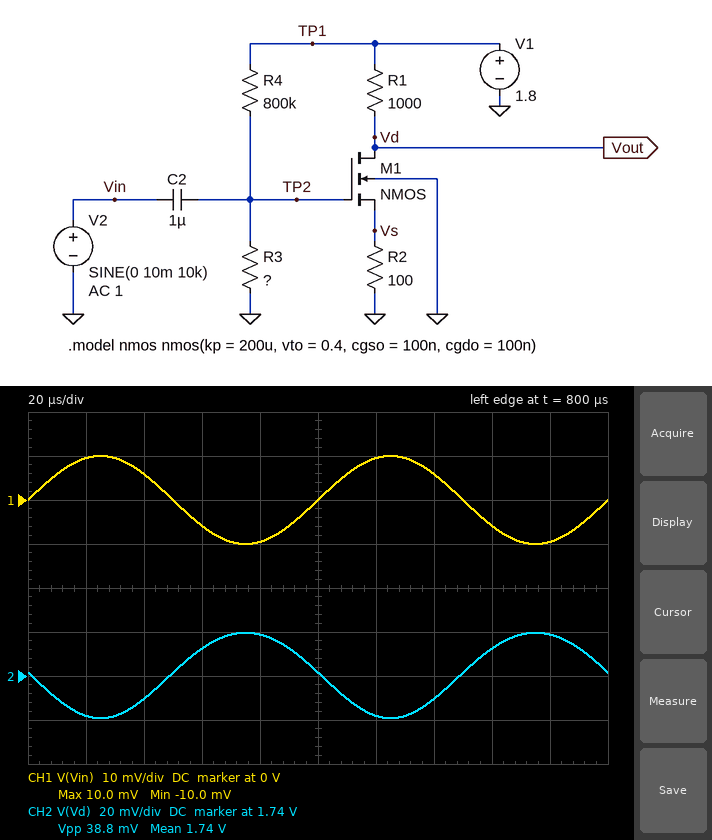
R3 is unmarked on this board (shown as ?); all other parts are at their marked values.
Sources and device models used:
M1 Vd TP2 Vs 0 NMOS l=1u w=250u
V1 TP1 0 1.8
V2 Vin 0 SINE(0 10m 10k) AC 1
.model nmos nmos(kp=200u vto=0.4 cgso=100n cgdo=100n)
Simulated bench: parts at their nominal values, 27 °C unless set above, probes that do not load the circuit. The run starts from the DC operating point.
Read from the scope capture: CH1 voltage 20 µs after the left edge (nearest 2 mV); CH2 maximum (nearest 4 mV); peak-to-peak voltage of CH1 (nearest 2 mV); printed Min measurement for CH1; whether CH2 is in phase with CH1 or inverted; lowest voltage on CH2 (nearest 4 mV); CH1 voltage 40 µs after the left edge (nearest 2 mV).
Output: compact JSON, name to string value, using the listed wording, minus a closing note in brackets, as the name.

{"CH1 voltage 20 µs after the left edge": "10 mV", "CH2 maximum": "1.760 V", "peak-to-peak voltage of CH1": "20 mV", "printed Min measurement for CH1": "-10.0 mV", "whether CH2 is in phase with CH1 or inverted": "inverted", "lowest voltage on CH2": "1.720 V", "CH1 voltage 40 µs after the left edge": "6 mV"}
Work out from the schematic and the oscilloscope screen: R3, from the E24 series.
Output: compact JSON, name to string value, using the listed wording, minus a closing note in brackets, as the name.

{"R3, from the E24 series": "270 kΩ"}
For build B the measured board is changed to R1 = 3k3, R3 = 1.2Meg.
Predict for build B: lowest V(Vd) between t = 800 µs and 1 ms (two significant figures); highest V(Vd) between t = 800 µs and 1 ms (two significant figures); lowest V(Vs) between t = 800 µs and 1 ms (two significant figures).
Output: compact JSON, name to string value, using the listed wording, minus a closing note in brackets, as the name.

{"lowest V(Vd) between t = 800 µs and 1 ms": "69 mV", "highest V(Vd) between t = 800 µs and 1 ms": "70 mV", "lowest V(Vs) between t = 800 µs and 1 ms": "52 mV"}
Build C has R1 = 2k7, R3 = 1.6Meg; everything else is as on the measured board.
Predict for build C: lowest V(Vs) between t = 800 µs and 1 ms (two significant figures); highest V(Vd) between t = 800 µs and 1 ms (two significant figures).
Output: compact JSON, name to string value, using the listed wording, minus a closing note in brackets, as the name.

{"lowest V(Vs) between t = 800 µs and 1 ms": "64 mV", "highest V(Vd) between t = 800 µs and 1 ms": "81 mV"}
